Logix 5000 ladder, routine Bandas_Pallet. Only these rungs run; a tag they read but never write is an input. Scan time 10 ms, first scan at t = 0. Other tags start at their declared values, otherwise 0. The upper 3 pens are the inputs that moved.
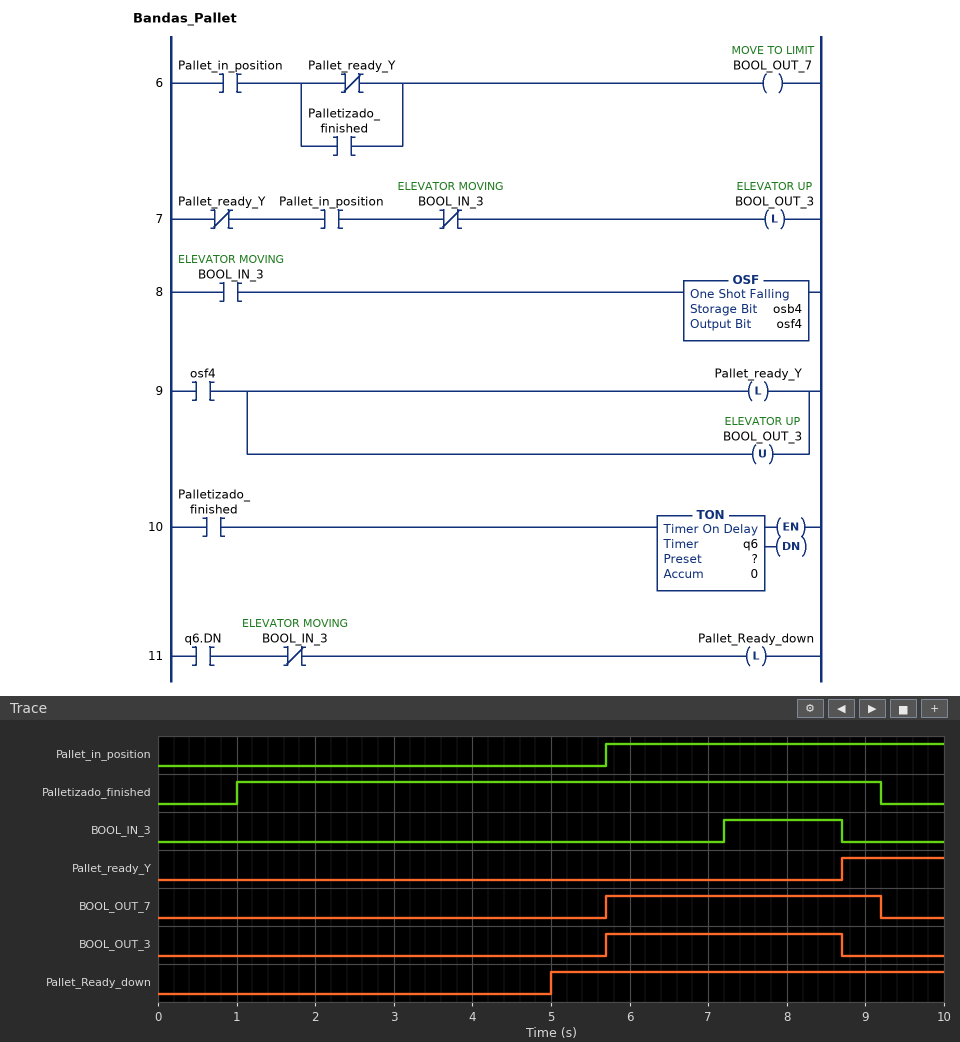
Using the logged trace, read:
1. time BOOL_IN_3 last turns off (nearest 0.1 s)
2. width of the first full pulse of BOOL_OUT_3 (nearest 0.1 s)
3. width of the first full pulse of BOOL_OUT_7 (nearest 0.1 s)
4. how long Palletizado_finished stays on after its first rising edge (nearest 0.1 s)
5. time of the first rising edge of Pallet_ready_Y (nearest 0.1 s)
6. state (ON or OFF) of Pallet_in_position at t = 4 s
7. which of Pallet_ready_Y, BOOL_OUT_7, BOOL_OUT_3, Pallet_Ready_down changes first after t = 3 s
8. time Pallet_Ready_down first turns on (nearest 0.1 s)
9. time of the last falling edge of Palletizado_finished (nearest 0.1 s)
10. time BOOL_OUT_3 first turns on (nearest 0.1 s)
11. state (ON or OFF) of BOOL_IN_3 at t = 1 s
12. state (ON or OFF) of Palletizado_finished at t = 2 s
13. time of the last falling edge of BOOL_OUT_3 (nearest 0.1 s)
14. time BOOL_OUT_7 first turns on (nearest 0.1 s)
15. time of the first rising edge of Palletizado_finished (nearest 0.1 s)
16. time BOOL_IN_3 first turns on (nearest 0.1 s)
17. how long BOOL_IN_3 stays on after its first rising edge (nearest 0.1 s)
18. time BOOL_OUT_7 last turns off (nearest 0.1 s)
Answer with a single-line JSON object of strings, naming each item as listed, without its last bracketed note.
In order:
{"time BOOL_IN_3 last turns off": "8.7 s", "width of the first full pulse of BOOL_OUT_3": "3.0 s", "width of the first full pulse of BOOL_OUT_7": "3.5 s", "how long Palletizado_finished stays on after its first rising edge": "8.2 s", "time of the first rising edge of Pallet_ready_Y": "8.7 s", "state (ON or OFF) of Pallet_in_position at t = 4 s": "OFF", "which of Pallet_ready_Y, BOOL_OUT_7, BOOL_OUT_3, Pallet_Ready_down changes first after t = 3 s": "Pallet_Ready_down", "time Pallet_Ready_down first turns on": "5.0 s", "time of the last falling edge of Palletizado_finished": "9.2 s", "time BOOL_OUT_3 first turns on": "5.7 s", "state (ON or OFF) of BOOL_IN_3 at t = 1 s": "OFF", "state (ON or OFF) of Palletizado_finished at t = 2 s": "ON", "time of the last falling edge of BOOL_OUT_3": "8.7 s", "time BOOL_OUT_7 first turns on": "5.7 s", "time of the first rising edge of Palletizado_finished": "1.0 s", "time BOOL_IN_3 first turns on": "7.2 s", "how long BOOL_IN_3 stays on after its first rising edge": "1.5 s", "time BOOL_OUT_7 last turns off": "9.2 s"}
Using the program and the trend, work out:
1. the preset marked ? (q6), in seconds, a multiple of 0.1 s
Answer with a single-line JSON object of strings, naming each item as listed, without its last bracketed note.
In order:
{"the preset marked ? (q6), in seconds, a multiple of 0.1 s": "4.0 s"}
